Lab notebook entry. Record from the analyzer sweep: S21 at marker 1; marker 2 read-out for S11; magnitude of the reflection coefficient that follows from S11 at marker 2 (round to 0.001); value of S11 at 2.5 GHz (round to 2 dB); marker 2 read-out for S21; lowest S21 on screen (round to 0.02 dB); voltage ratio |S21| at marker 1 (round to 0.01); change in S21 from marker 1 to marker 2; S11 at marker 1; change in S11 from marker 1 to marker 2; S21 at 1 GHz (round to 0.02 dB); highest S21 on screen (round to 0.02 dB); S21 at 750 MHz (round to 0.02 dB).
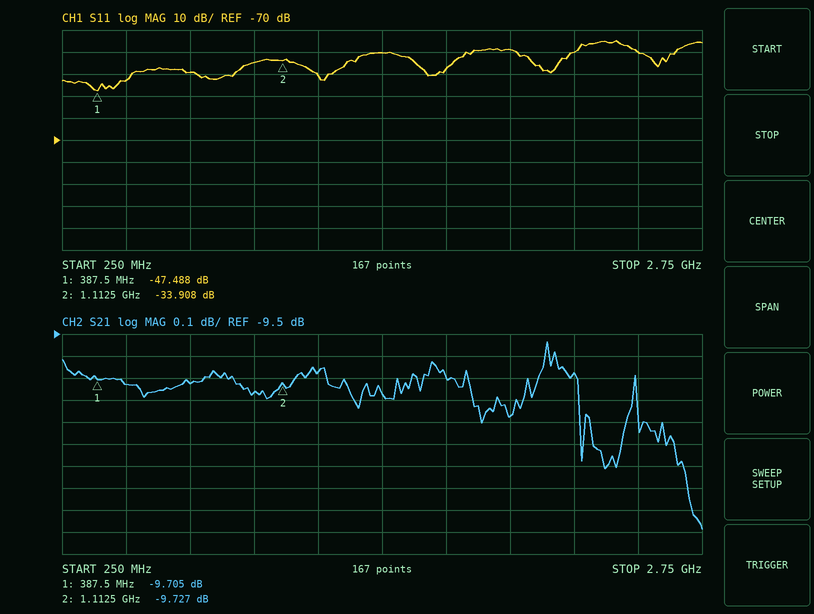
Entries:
-9.705 dB
-33.908 dB
0.020
-30 dB
-9.727 dB
-10.38 dB
0.33
-0.022 dB
-47.488 dB
13.580 dB
-9.76 dB
-9.54 dB
-9.72 dB
